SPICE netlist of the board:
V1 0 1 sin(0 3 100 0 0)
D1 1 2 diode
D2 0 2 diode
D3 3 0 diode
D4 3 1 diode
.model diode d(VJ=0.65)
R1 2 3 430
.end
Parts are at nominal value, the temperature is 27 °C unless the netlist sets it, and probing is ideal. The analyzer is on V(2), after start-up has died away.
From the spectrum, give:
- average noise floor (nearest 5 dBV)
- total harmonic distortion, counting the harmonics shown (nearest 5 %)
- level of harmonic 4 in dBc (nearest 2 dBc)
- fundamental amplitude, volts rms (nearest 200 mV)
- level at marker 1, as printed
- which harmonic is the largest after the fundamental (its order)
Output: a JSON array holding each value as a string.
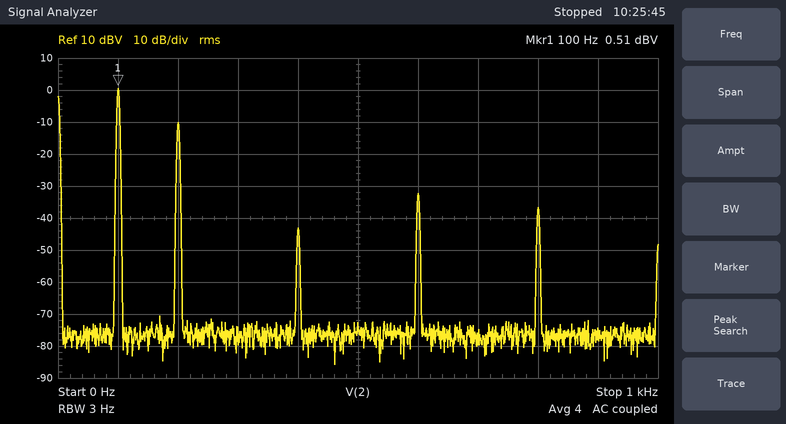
["-75 dBV", "30 %", "-44 dBc", "1.0 V", "0.51 dBV", "2"]
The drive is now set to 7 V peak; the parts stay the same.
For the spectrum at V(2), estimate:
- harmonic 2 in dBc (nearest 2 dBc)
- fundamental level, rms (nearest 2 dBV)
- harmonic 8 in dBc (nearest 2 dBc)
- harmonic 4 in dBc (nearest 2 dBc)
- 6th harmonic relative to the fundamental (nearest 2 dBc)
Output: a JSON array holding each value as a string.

["-8 dBc", "8 dBV", "-56 dBc", "-24 dBc", "-36 dBc"]
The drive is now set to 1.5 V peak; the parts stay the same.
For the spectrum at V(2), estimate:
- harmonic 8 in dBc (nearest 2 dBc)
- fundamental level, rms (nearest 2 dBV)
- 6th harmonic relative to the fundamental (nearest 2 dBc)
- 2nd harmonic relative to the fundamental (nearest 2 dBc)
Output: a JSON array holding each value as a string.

["-50 dBc", "-6 dBV", "-42 dBc", "-24 dBc"]
